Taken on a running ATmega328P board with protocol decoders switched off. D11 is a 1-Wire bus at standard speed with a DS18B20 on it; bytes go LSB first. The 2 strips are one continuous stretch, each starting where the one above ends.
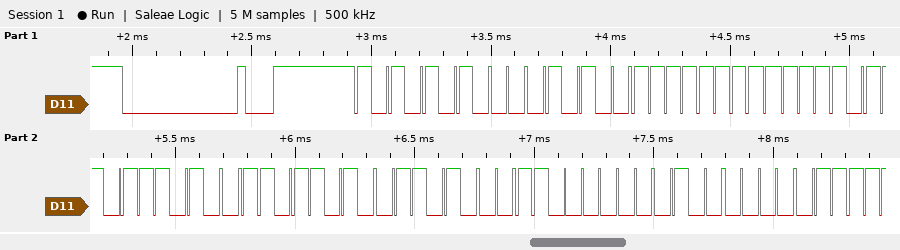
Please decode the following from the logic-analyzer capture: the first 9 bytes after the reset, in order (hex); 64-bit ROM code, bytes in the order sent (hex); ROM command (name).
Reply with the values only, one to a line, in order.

55 28 FF DF 2E 5B 16 03 02
28 FF DF 2E 5B 16 03 02
Match ROM
